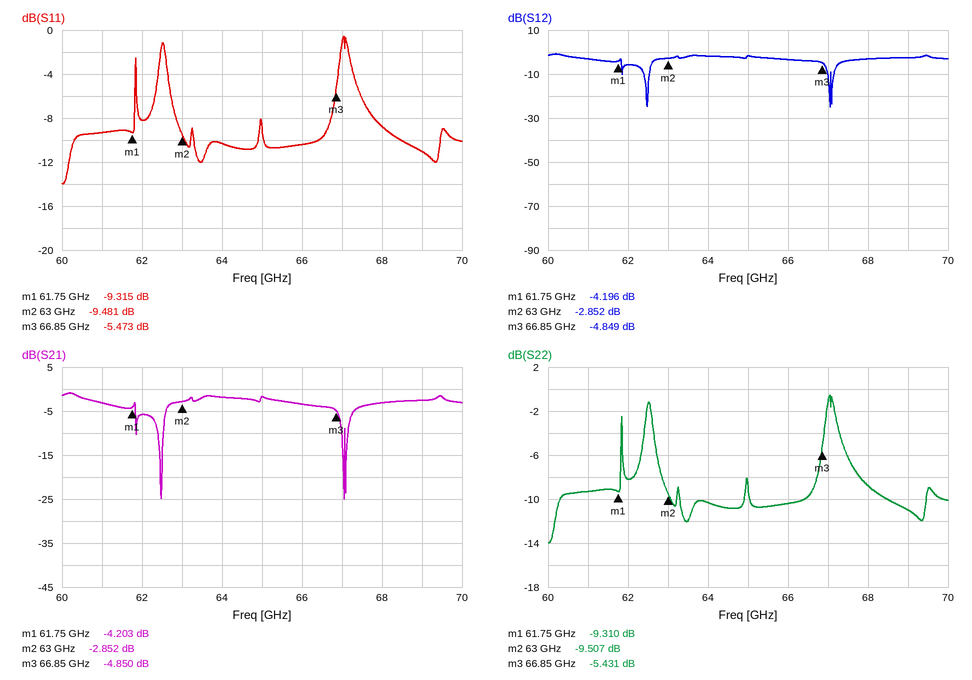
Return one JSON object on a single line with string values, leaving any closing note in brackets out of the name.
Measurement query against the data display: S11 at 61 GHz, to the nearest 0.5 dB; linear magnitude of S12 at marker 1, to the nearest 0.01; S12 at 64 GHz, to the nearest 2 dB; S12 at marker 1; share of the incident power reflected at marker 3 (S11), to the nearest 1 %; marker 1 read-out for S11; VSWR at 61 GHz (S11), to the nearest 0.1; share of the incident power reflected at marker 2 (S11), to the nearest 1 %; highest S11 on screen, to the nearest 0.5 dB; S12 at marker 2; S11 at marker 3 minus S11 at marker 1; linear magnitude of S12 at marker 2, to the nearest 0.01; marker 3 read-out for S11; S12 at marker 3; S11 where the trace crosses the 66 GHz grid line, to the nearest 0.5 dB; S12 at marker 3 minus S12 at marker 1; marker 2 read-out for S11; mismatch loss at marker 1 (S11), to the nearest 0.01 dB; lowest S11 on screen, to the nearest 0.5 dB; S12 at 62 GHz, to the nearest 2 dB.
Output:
{"S11 at 61 GHz, to the nearest 0.5 dB": "-9.5 dB", "linear magnitude of S12 at marker 1, to the nearest 0.01": "0.62", "S12 at 64 GHz, to the nearest 2 dB": "-2 dB", "S12 at marker 1": "-4.196 dB", "share of the incident power reflected at marker 3 (S11), to the nearest 1 %": "28 %", "marker 1 read-out for S11": "-9.315 dB", "VSWR at 61 GHz (S11), to the nearest 0.1": "2.0", "share of the incident power reflected at marker 2 (S11), to the nearest 1 %": "11 %", "highest S11 on screen, to the nearest 0.5 dB": "-0.5 dB", "S12 at marker 2": "-2.852 dB", "S11 at marker 3 minus S11 at marker 1": "3.842 dB", "linear magnitude of S12 at marker 2, to the nearest 0.01": "0.72", "marker 3 read-out for S11": "-5.473 dB", "S12 at marker 3": "-4.849 dB", "S11 where the trace crosses the 66 GHz grid line, to the nearest 0.5 dB": "-10.5 dB", "S12 at marker 3 minus S12 at marker 1": "-0.653 dB", "marker 2 read-out for S11": "-9.481 dB", "mismatch loss at marker 1 (S11), to the nearest 0.01 dB": "0.54 dB", "lowest S11 on screen, to the nearest 0.5 dB": "-14.0 dB", "S12 at 62 GHz, to the nearest 2 dB": "-6 dB"}
